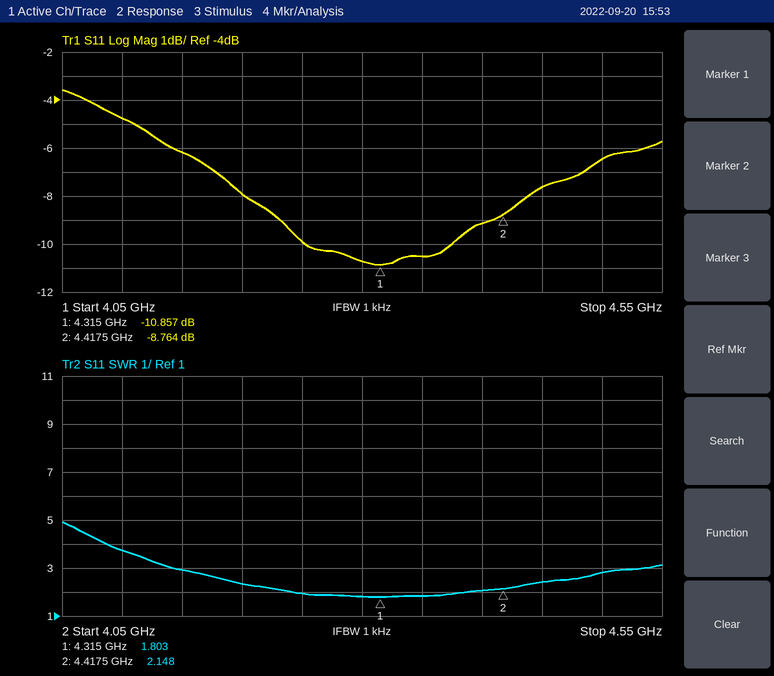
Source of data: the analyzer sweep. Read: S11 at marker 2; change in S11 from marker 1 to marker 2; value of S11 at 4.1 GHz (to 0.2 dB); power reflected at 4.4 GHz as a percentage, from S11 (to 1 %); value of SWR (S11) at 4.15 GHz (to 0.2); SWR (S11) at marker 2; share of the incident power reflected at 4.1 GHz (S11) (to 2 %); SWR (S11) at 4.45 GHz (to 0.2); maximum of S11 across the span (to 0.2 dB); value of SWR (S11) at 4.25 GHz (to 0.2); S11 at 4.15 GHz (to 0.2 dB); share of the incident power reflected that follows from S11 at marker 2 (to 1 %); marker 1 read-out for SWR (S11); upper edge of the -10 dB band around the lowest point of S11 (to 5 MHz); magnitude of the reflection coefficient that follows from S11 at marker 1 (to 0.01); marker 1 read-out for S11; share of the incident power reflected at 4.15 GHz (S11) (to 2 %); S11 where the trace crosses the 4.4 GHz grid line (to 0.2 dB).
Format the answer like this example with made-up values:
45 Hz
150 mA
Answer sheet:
-8.764 dB
2.093 dB
-4.8 dB
12 %
3.0
2.148
34 %
2.4
-3.6 dB
2.0
-6.2 dB
13 %
1.803
4.375 GHz
0.29
-10.857 dB
24 %
-9.2 dB
